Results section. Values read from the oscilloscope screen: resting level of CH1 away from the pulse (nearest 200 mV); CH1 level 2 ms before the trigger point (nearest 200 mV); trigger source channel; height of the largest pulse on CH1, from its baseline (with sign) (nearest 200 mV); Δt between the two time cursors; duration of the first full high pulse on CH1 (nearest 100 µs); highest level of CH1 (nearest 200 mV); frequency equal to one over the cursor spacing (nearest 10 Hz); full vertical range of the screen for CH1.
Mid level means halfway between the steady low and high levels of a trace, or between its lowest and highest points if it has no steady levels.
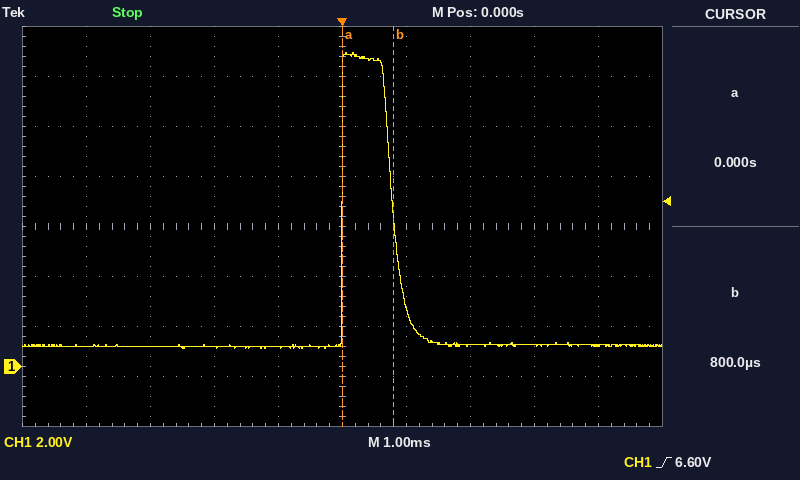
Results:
800 mV
800 mV
CH1
+11.8 V
800 µs
800 µs
12.6 V
1.25 kHz
16 V
